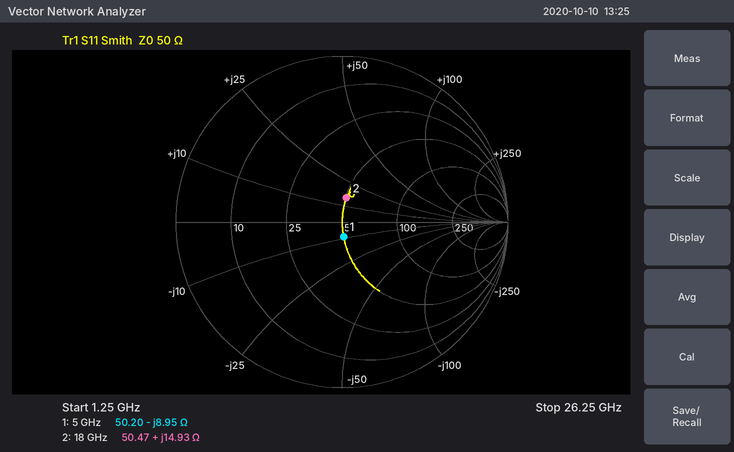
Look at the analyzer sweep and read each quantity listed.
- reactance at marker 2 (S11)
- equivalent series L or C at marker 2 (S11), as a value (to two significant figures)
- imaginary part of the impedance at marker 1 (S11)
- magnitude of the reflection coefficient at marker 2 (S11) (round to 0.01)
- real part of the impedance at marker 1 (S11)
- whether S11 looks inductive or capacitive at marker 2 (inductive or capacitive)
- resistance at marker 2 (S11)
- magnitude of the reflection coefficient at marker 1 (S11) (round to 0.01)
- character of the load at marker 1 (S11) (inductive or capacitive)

+14.93 Ω
130 pH
-8.95 Ω
0.15
50.20 Ω
inductive
50.47 Ω
0.09
capacitive
